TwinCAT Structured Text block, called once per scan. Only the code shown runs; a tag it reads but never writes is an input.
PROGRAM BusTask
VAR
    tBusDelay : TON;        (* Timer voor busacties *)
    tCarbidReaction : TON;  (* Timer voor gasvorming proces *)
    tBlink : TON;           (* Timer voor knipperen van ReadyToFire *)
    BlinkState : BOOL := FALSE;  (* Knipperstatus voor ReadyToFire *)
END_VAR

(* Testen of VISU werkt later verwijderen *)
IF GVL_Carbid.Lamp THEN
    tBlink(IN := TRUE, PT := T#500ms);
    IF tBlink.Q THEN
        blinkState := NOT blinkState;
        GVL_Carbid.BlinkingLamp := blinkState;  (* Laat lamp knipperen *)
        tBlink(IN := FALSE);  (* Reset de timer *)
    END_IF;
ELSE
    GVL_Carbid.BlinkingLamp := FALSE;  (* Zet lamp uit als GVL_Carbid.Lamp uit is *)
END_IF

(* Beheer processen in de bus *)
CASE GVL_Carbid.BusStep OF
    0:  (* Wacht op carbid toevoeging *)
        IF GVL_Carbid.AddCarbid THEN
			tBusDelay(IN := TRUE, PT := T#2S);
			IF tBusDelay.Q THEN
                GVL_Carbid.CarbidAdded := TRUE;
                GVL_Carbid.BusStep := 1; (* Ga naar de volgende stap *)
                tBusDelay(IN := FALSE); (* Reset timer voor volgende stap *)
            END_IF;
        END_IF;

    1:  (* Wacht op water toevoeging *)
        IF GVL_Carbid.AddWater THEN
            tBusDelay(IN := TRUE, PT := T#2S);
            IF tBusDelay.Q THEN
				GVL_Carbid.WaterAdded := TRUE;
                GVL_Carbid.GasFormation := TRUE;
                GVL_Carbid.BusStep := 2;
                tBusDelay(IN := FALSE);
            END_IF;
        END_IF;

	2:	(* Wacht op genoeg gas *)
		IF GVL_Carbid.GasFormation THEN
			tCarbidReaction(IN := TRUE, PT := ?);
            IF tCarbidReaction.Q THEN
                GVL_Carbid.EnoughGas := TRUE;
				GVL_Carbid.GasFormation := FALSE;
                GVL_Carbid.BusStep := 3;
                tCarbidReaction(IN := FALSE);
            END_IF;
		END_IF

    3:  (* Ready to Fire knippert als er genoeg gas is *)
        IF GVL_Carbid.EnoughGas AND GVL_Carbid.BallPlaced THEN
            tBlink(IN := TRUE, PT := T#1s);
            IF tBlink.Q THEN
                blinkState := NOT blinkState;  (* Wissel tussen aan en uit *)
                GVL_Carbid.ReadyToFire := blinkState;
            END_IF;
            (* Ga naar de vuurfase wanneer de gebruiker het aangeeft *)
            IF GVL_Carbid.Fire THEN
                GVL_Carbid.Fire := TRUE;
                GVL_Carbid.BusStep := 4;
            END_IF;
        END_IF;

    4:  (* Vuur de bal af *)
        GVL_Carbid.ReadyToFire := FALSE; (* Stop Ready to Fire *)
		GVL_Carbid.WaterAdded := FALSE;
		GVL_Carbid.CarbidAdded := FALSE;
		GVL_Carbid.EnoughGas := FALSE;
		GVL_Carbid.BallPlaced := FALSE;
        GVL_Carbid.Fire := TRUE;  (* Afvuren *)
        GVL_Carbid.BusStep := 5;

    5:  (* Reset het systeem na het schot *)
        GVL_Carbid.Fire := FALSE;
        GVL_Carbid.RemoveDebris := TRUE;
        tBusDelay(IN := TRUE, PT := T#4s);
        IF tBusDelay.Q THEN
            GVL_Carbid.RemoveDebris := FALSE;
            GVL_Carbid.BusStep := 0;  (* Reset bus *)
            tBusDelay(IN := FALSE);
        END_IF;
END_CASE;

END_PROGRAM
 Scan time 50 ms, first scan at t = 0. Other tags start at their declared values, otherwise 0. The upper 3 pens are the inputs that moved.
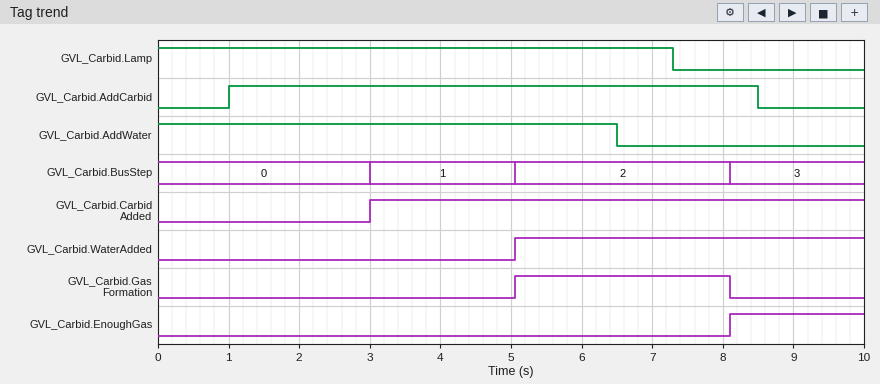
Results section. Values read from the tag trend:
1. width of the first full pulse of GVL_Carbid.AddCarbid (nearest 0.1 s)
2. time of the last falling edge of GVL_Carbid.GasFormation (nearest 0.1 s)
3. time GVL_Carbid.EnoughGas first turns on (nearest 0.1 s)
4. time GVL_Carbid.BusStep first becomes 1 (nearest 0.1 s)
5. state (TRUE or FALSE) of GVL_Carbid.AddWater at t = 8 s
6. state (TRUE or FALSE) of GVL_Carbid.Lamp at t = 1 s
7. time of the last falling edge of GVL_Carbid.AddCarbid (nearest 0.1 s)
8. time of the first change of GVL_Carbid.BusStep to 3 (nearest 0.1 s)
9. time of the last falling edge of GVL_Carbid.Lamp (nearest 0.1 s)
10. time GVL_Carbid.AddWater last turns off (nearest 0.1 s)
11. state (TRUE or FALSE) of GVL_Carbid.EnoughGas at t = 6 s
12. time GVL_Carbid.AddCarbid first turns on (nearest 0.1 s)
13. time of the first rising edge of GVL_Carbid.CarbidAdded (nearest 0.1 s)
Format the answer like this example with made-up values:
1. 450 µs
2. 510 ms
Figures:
1. 7.5 s
2. 8.1 s
3. 8.1 s
4. 3.0 s
5. FALSE
6. TRUE
7. 8.5 s
8. 8.1 s
9. 7.3 s
10. 6.5 s
11. FALSE
12. 1.0 s
13. 3.0 s
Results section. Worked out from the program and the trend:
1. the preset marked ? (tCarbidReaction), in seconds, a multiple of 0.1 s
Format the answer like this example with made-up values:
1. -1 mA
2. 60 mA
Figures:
1. 3.0 s
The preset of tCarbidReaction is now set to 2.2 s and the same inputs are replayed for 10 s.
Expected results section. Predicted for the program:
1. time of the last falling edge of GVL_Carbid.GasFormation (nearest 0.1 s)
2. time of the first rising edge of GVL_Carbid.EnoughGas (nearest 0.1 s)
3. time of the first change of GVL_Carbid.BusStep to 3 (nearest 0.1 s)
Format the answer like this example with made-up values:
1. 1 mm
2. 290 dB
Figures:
1. 7.3 s
2. 7.3 s
3. 7.3 s
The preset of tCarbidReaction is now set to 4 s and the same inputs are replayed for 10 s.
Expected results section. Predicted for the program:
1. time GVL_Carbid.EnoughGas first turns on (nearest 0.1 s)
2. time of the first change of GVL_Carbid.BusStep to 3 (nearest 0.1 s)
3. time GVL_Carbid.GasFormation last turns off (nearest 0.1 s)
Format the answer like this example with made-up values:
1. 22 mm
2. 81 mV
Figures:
1. 9.1 s
2. 9.1 s
3. 9.1 s
